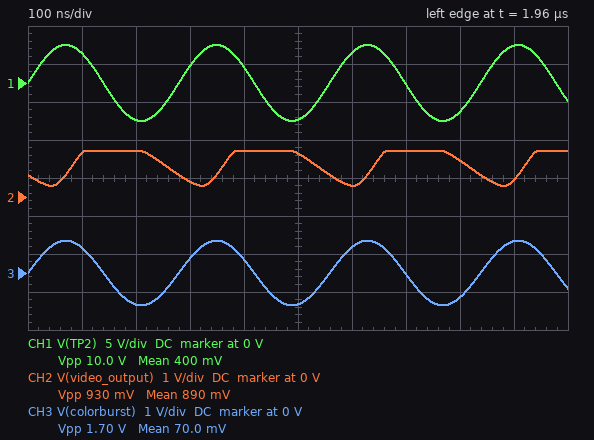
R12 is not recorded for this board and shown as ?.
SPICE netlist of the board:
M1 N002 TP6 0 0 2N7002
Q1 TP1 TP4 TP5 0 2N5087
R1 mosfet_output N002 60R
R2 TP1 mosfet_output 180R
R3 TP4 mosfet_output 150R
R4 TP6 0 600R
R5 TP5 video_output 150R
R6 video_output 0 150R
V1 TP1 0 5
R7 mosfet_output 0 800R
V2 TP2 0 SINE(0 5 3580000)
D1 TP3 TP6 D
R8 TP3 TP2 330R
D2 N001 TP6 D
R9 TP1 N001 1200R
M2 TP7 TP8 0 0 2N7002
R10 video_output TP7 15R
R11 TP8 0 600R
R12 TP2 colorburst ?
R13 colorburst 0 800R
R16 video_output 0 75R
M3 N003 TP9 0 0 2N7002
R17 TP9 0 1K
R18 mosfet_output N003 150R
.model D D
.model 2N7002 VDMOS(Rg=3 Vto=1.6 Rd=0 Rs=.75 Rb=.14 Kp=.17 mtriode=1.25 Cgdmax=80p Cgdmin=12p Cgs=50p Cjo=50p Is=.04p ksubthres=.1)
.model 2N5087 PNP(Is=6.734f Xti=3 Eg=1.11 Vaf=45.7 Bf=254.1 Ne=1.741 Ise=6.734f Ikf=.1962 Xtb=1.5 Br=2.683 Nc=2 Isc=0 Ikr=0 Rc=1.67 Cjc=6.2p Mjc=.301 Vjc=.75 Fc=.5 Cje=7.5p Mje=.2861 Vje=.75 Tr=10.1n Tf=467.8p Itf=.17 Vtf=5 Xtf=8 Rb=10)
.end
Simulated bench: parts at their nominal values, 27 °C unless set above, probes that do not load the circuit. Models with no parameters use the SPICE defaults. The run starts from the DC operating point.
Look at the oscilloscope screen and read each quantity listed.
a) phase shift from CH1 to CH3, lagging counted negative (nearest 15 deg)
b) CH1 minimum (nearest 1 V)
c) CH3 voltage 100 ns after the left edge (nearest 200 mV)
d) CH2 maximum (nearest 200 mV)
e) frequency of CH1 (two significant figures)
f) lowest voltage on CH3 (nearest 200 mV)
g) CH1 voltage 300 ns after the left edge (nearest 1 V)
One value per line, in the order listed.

0 deg
-5 V
600 mV
1.2 V
3.6 MHz
-800 mV
2 V
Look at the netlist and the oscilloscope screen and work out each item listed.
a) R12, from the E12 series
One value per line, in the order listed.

3.9 kΩ
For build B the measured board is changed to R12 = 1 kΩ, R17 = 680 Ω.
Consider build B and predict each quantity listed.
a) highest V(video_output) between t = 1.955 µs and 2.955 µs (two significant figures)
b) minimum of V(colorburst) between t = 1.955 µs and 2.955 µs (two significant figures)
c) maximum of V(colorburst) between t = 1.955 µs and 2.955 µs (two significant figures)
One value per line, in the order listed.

1.2 V
-2.2 V
2.2 V
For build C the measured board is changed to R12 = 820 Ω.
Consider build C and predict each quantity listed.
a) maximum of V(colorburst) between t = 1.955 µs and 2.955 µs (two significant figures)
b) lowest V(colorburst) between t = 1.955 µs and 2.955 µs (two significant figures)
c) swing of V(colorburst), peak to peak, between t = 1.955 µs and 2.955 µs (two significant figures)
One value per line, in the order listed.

2.5 V
-2.5 V
4.9 V
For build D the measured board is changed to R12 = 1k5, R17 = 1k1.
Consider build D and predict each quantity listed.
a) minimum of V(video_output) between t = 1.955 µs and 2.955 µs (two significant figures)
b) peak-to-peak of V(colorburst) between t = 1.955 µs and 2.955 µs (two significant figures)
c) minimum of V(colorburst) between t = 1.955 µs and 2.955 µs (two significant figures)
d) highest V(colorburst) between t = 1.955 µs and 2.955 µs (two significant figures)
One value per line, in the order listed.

290 mV
3.5 V
-1.7 V
1.7 V
